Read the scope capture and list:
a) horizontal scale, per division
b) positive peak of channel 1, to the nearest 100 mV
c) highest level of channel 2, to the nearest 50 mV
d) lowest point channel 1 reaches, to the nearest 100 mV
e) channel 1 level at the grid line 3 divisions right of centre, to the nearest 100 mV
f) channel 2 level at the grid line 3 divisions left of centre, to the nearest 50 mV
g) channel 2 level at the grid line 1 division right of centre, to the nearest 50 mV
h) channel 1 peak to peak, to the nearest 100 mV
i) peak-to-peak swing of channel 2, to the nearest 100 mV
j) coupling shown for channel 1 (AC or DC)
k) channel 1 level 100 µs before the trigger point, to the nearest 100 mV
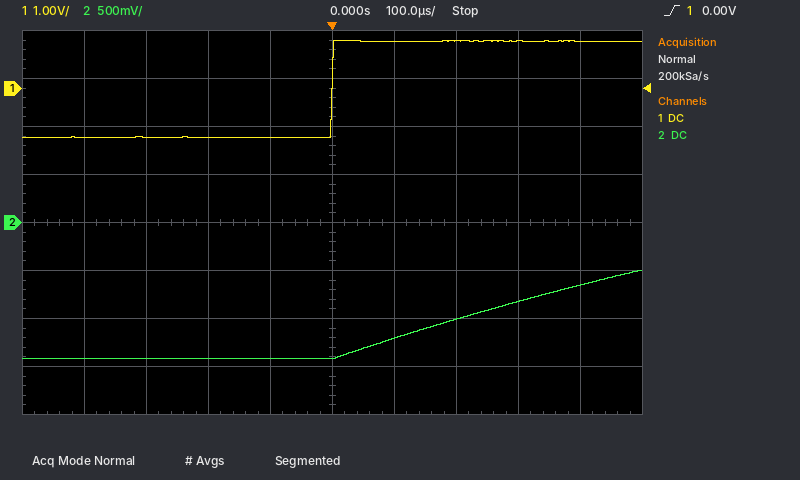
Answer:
100 µs
1.0 V
-500 mV
-1.0 V
1.0 V
-1.40 V
-1.20 V
2.0 V
900 mV
DC
-1.0 V
